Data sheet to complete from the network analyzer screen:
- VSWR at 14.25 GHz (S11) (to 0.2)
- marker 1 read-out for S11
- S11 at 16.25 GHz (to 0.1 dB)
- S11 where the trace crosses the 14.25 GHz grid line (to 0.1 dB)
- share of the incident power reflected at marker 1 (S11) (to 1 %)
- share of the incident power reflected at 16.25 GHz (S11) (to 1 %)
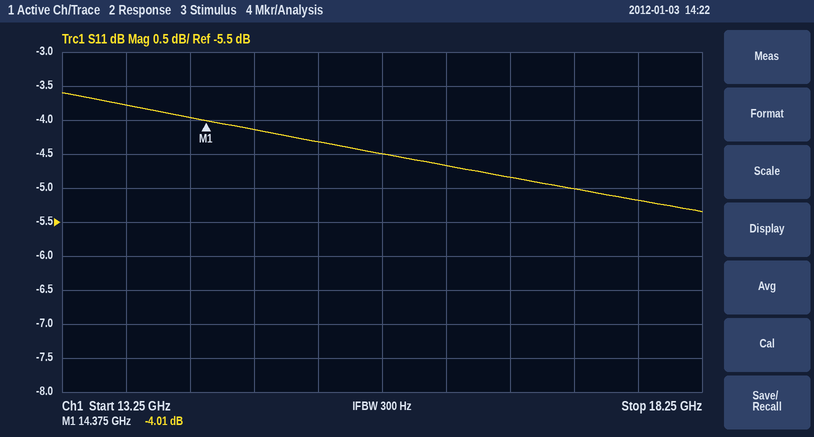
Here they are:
4.4
-4.01 dB
-4.7 dB
-4.0 dB
40 %
34 %
